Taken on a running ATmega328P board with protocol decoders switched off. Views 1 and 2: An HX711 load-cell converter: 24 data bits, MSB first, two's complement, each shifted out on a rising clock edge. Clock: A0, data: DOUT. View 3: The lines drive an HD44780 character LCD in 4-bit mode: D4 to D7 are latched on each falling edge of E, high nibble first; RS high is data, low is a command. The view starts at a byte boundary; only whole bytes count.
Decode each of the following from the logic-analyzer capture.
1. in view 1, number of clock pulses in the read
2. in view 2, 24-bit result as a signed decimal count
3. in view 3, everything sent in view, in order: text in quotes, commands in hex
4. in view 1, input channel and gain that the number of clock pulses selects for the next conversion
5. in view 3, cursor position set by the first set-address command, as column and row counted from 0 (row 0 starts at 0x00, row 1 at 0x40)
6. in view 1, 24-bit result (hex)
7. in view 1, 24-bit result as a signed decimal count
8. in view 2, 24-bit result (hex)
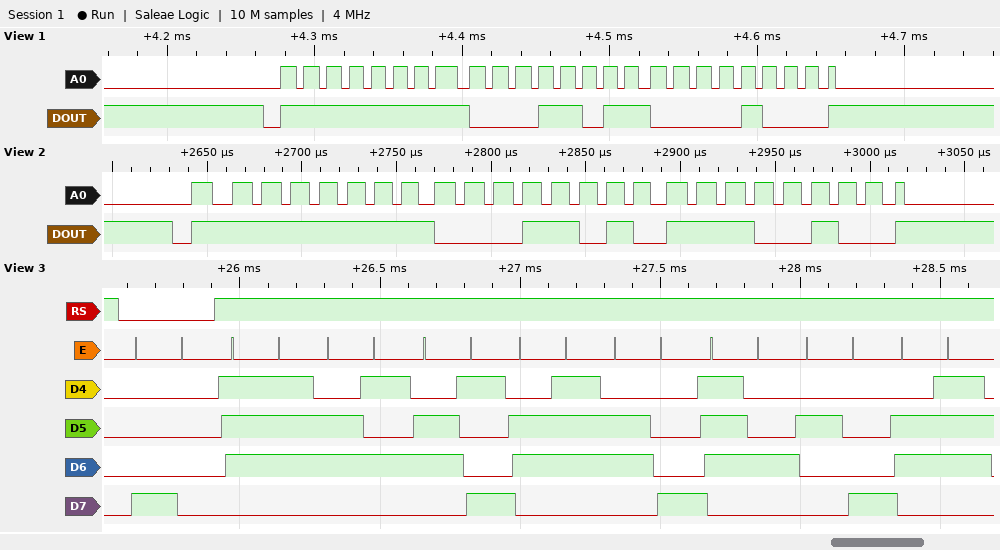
25
-58652
0x80 "weight(g"
channel A, gain 128
column 0, row 0
0xFF1B08
-58616
0xFF1AE4
